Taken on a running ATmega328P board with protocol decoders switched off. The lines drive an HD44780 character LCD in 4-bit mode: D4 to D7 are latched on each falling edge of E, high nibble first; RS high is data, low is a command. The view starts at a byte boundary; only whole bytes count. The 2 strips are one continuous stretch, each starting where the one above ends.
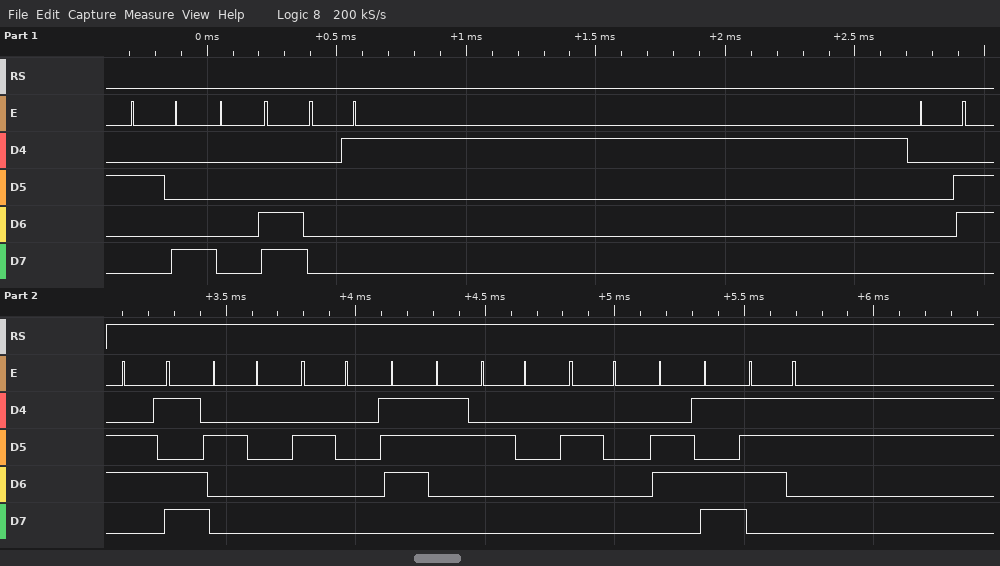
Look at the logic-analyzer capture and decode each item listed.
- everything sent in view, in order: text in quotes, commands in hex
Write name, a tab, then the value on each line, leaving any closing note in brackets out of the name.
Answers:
everything sent in view, in order: text in quotes, commands in hex	0x28 0x0C 0x01 0x06 "m  s  ms"
